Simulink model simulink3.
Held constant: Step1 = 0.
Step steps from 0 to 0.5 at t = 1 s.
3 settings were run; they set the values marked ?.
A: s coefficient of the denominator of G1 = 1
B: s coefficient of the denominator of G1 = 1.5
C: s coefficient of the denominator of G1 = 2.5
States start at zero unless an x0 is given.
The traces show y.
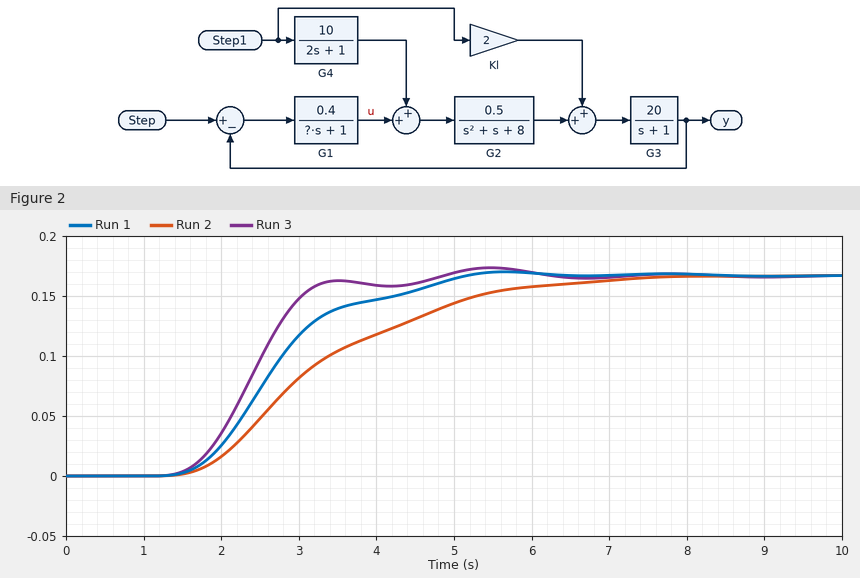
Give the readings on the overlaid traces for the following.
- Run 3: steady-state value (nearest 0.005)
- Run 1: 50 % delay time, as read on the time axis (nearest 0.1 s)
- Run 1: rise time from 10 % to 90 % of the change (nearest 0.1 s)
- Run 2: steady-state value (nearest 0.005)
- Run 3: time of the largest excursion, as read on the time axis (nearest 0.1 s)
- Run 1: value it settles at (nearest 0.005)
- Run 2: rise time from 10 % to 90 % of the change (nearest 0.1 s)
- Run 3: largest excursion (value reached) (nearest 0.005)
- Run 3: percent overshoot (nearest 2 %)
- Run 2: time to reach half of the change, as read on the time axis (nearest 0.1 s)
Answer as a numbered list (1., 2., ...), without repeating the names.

1. 0.165
2. 2.6 s
3. 2.4 s
4. 0.165
5. 5.5 s
6. 0.165
7. 3.3 s
8. 0.175
9. 4 %
10. 3.0 s
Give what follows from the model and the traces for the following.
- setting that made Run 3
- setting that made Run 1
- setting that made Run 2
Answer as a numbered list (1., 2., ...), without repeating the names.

1. A
2. B
3. C
